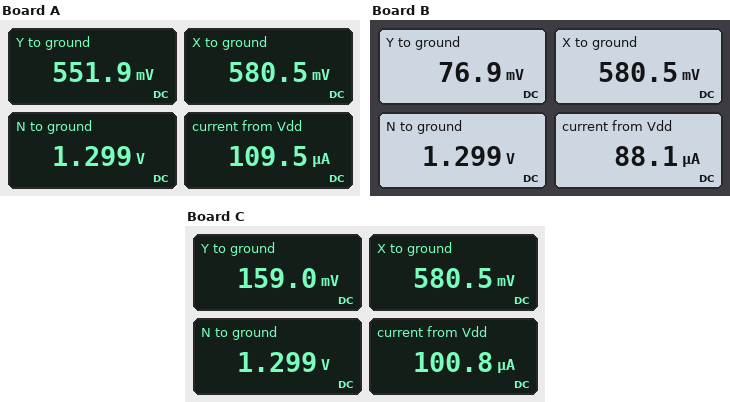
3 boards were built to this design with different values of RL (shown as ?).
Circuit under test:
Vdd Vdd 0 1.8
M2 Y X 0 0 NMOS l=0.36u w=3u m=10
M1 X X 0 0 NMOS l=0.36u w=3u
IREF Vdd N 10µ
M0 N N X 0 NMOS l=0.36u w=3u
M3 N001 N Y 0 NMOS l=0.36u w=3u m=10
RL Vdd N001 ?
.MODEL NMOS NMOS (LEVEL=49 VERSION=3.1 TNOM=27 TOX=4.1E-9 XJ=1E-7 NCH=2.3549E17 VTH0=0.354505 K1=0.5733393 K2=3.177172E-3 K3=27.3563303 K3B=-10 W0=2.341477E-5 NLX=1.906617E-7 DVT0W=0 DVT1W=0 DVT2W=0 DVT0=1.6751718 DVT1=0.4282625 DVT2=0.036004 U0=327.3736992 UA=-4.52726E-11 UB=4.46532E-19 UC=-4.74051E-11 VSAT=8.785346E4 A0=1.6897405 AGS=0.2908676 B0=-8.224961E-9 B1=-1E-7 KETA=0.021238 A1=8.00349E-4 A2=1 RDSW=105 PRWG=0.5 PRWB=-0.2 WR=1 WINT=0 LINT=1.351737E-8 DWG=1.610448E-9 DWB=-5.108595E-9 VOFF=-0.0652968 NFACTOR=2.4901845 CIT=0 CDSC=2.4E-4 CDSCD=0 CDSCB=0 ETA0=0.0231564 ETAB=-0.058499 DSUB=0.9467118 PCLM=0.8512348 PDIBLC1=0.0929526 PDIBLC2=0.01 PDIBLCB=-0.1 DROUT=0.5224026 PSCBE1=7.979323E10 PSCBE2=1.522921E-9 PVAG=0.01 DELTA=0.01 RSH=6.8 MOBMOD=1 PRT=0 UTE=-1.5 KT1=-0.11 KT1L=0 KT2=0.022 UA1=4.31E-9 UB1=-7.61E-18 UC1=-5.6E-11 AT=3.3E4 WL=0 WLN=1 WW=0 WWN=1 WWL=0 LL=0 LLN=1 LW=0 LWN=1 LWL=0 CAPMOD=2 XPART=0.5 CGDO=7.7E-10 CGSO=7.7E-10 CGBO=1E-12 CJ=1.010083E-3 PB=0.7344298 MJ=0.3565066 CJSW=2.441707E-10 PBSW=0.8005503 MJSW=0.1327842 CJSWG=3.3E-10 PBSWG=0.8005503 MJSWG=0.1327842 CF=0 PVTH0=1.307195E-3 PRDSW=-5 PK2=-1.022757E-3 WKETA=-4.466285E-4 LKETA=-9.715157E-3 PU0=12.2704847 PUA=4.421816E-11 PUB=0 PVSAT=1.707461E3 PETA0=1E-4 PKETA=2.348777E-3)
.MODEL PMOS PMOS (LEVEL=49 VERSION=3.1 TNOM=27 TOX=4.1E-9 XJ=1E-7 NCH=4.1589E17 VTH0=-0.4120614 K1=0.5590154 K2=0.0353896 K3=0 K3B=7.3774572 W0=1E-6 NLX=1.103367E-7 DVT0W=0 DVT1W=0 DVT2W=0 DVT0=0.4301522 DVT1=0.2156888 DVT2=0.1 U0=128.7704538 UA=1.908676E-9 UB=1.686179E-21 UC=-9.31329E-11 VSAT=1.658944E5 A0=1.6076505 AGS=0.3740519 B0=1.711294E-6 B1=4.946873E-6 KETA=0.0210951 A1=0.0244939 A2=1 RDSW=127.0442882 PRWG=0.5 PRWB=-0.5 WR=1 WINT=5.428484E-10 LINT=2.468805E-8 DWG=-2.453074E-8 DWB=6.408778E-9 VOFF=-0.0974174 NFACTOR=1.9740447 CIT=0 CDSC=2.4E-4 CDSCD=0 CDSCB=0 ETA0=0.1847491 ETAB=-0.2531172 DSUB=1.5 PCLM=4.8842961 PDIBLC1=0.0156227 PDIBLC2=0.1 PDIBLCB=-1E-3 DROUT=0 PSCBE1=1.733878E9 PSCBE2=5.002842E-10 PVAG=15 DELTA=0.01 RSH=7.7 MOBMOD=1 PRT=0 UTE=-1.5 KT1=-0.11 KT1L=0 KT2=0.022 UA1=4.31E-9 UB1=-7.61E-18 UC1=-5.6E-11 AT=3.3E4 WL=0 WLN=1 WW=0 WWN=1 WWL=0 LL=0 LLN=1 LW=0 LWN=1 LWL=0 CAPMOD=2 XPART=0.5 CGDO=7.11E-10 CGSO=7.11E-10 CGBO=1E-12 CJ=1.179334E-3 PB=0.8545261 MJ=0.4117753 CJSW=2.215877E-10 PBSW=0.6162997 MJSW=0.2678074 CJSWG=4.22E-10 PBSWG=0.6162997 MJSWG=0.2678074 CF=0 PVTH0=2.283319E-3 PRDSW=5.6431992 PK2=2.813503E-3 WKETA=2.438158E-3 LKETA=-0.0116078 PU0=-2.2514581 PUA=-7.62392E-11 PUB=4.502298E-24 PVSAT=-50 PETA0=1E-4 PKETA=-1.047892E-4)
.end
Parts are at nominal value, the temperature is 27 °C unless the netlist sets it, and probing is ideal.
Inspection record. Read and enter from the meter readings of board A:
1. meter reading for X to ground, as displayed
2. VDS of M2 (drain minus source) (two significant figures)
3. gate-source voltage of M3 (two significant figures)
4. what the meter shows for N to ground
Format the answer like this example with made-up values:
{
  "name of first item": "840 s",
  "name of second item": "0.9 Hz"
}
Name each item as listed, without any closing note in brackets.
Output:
{
  "meter reading for X to ground, as displayed": "580.5 mV",
  "VDS of M2 (drain minus source)": "550 mV",
  "gate-source voltage of M3": "750 mV",
  "what the meter shows for N to ground": "1.299 V"
}
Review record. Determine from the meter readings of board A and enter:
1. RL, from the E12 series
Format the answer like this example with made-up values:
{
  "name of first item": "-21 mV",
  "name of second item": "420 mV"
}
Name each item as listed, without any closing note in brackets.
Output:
{
  "RL, from the E12 series": "12 kΩ"
}
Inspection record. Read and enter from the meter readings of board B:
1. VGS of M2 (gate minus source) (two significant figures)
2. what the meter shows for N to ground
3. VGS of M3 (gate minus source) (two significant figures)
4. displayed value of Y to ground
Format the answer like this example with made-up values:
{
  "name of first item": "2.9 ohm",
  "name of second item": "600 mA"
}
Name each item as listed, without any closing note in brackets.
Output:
{
  "VGS of M2 (gate minus source)": "580 mV",
  "what the meter shows for N to ground": "1.299 V",
  "VGS of M3 (gate minus source)": "1.2 V",
  "displayed value of Y to ground": "76.9 mV"
}
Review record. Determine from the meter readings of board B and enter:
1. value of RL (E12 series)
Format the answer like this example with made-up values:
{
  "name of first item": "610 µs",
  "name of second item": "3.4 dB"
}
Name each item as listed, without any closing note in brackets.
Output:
{
  "value of RL": "22 kΩ"
}
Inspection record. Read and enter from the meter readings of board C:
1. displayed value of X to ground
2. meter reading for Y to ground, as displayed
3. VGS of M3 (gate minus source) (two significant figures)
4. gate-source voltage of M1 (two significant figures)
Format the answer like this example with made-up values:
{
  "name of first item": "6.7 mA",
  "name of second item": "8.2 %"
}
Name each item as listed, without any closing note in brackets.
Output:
{
  "displayed value of X to ground": "580.5 mV",
  "meter reading for Y to ground, as displayed": "159.0 mV",
  "VGS of M3 (gate minus source)": "1.1 V",
  "gate-source voltage of M1": "580 mV"
}
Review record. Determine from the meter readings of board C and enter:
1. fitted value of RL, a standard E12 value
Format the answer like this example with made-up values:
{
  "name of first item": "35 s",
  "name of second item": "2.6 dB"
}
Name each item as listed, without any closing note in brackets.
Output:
{
  "fitted value of RL, a standard E12 value": "18 kΩ"
}
